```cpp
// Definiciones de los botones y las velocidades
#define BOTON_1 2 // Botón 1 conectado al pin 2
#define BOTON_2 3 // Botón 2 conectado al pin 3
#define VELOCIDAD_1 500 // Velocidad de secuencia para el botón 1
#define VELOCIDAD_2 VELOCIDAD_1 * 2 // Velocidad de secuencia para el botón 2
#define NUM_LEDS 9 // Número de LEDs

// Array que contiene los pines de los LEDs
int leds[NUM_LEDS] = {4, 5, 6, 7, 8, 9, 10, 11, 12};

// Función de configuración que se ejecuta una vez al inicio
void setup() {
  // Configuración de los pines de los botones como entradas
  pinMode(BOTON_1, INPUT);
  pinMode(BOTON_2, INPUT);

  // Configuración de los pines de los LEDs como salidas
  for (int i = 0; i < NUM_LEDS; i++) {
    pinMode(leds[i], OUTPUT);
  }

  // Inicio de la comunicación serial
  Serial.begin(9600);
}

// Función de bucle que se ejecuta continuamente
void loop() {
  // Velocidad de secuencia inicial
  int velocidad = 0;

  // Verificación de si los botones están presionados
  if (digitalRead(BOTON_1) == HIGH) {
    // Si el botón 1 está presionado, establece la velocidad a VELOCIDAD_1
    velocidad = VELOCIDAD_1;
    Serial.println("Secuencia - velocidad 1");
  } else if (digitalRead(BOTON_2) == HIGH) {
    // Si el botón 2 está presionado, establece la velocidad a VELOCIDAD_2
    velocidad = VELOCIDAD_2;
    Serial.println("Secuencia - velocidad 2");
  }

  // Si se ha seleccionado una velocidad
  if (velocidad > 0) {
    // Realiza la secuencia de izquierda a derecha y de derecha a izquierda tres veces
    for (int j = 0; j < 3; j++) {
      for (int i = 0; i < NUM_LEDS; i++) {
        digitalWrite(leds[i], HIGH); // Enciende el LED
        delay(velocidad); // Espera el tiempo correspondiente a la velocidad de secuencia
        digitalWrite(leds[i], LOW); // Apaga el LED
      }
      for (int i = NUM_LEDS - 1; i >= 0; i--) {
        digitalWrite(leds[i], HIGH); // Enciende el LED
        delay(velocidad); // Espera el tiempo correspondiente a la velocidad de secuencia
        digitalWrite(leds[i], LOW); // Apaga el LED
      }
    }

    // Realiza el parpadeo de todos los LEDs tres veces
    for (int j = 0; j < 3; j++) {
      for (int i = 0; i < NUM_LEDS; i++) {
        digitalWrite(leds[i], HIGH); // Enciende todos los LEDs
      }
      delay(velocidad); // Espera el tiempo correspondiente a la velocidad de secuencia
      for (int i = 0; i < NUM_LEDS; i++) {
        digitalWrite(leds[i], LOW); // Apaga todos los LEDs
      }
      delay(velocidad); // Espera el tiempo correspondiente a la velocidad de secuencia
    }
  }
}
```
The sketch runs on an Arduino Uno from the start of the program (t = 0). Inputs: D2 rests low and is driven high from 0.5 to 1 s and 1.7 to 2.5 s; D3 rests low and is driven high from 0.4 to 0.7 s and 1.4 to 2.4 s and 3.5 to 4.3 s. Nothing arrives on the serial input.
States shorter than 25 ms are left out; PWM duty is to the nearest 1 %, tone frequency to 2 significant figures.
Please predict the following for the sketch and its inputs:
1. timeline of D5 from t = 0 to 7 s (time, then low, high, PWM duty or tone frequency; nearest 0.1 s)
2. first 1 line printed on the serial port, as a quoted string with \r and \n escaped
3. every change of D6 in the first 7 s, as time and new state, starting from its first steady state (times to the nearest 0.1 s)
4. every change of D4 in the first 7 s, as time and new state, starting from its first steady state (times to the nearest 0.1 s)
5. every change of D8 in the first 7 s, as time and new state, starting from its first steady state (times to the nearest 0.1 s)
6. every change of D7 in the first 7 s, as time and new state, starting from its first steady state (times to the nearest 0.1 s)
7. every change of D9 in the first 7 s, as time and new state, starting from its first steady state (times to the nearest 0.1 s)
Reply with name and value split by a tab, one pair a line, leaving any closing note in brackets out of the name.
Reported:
timeline of D5 from t = 0 to 7 s	0 s low; 1.4 s high; 2.4 s low
first 1 line printed on the serial port, as a quoted string with \r and \n escaped	"Secuencia - velocidad 2\r\n"
every change of D6 in the first 7 s, as time and new state, starting from its first steady state	0 s low; 2.4 s high; 3.4 s low
every change of D4 in the first 7 s, as time and new state, starting from its first steady state	0 s low; 0.4 s high; 1.4 s low
every change of D8 in the first 7 s, as time and new state, starting from its first steady state	0 s low; 4.4 s high; 5.4 s low
every change of D7 in the first 7 s, as time and new state, starting from its first steady state	0 s low; 3.4 s high; 4.4 s low
every change of D9 in the first 7 s, as time and new state, starting from its first steady state	0 s low; 5.4 s high; 6.4 s low
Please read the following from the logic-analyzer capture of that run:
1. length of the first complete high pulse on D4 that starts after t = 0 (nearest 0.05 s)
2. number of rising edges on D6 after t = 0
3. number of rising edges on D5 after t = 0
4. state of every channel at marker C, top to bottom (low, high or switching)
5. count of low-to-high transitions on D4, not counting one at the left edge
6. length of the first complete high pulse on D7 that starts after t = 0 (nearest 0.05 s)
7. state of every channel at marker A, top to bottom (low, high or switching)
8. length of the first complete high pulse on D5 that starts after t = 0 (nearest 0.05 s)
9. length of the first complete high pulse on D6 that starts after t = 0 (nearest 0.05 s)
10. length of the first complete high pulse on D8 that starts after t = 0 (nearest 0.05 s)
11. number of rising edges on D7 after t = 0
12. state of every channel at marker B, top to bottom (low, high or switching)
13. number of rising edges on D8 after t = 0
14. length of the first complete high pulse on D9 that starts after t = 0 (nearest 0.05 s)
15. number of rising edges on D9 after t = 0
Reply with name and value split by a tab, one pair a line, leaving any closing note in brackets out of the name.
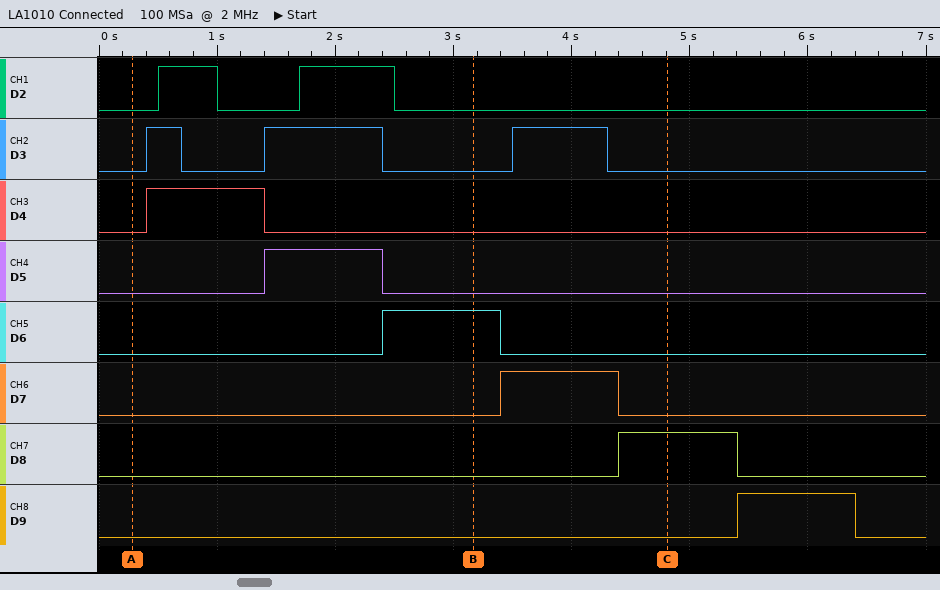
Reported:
length of the first complete high pulse on D4 that starts after t = 0	1.00 s
number of rising edges on D6 after t = 0	1
number of rising edges on D5 after t = 0	1
state of every channel at marker C, top to bottom	D2 low, D3 low, D4 low, D5 low, D6 low, D7 low, D8 high, D9 low
count of low-to-high transitions on D4, not counting one at the left edge	1
length of the first complete high pulse on D7 that starts after t = 0	1.00 s
state of every channel at marker A, top to bottom	D2 low, D3 low, D4 low, D5 low, D6 low, D7 low, D8 low, D9 low
length of the first complete high pulse on D5 that starts after t = 0	1.00 s
length of the first complete high pulse on D6 that starts after t = 0	1.00 s
length of the first complete high pulse on D8 that starts after t = 0	1.00 s
number of rising edges on D7 after t = 0	1
state of every channel at marker B, top to bottom	D2 low, D3 low, D4 low, D5 low, D6 high, D7 low, D8 low, D9 low
number of rising edges on D8 after t = 0	1
length of the first complete high pulse on D9 that starts after t = 0	1.00 s
number of rising edges on D9 after t = 0	1
